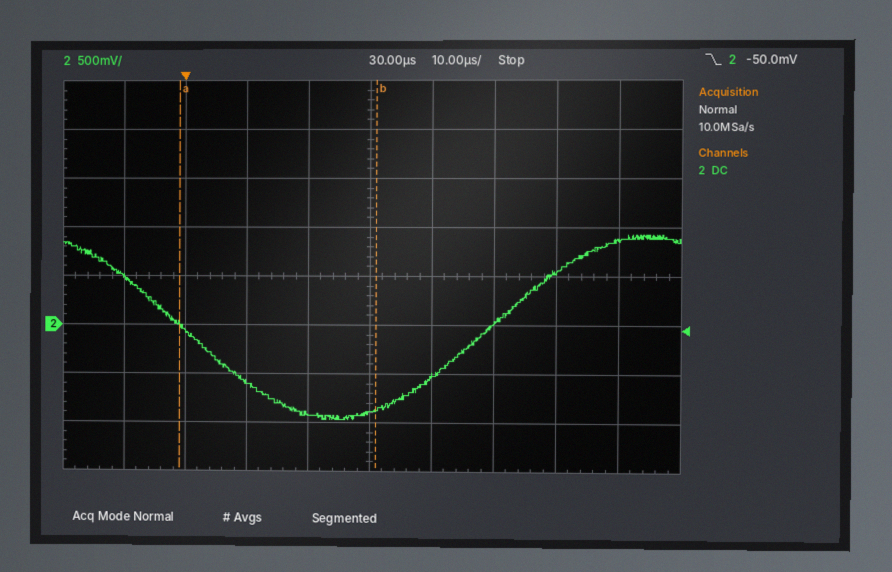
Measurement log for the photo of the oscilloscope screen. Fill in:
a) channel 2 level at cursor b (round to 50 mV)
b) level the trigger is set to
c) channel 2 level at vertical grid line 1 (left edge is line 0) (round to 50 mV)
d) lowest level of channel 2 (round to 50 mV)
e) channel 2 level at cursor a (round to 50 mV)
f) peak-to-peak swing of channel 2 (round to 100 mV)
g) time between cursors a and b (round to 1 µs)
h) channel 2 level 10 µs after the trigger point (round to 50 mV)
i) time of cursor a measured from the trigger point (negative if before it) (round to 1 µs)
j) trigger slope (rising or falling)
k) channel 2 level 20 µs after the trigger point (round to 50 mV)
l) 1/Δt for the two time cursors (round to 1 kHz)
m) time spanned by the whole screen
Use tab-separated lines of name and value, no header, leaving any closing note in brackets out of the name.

channel 2 level at cursor b	-850 mV
level the trigger is set to	-50.0 mV
channel 2 level at vertical grid line 1 (left edge is line 0)	500 mV
lowest level of channel 2	-950 mV
channel 2 level at cursor a	0 mV
peak-to-peak swing of channel 2	1.90 V
time between cursors a and b	32 µs
channel 2 level 10 µs after the trigger point	-600 mV
time of cursor a measured from the trigger point (negative if before it)	-1 µs
trigger slope	falling
channel 2 level 20 µs after the trigger point	-900 mV
1/Δt for the two time cursors	31 kHz
time spanned by the whole screen	100 µs
